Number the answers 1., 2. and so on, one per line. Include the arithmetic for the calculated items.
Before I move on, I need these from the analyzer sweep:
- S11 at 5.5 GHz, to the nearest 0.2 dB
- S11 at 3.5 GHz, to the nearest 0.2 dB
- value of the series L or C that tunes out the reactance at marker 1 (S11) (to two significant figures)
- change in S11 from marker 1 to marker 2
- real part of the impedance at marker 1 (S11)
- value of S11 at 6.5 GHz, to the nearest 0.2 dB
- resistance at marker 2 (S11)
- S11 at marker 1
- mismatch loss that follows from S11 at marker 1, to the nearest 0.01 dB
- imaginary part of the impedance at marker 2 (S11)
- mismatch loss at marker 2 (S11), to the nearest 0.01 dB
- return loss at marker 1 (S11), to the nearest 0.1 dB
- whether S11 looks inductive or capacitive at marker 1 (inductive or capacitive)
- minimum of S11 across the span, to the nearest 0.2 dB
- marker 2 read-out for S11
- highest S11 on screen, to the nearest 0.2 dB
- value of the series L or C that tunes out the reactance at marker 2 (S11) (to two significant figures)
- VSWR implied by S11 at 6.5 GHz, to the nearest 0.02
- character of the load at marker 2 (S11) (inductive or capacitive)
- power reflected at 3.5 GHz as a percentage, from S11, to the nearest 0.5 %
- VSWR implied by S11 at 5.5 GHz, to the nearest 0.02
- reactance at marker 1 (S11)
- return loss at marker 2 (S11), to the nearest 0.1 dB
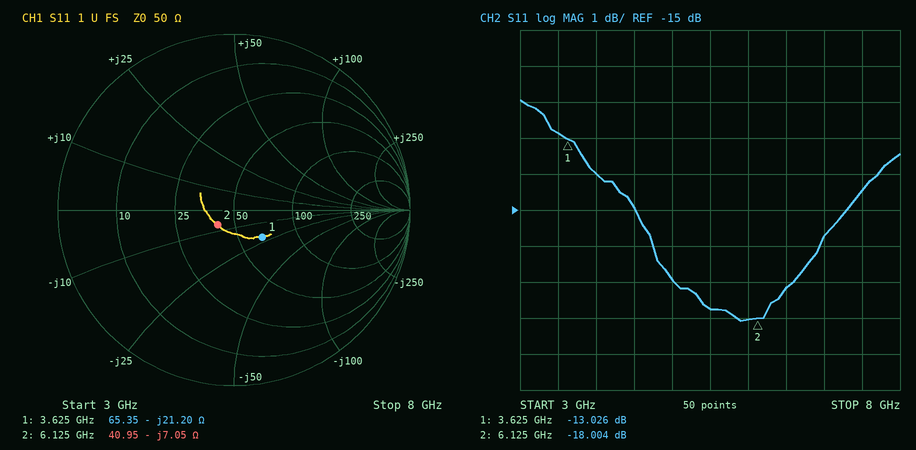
1. -17.8 dB
2. -12.8 dB
3. L = 21.2 Ω/(2π × 3.625 GHz) ≈ 931 pH, so 930 pH to two significant figures
4. -18.004 − (-13.026) = -4.978 dB
5. 65.35 Ω
6. -17.2 dB
7. 40.95 Ω
8. -13.026 dB
9. −10 log10(1 − 10^(-13.026/10)) ≈ 0.22 dB
10. -7.05 Ω
11. −10 log10(1 − 10^(-18.004/10)) ≈ 0.07 dB
12. 13.0 dB
13. capacitive
14. -18.0 dB
15. -18.004 dB
16. -12.0 dB
17. L = 7.05 Ω/(2π × 6.125 GHz) ≈ 183 pH, so 180 pH to two significant figures
18. |Γ| = 10^(-17.2/20) = 0.1380; VSWR = (1 + 0.1380)/(1 − 0.1380) ≈ 1.32
19. capacitive
20. 10^(-12.8/10) ≈ 5.25 %, so 5.0 % to the nearest 0.5 %
21. |Γ| = 10^(-17.8/20) = 0.1288; VSWR = (1 + 0.1288)/(1 − 0.1288) ≈ 1.30
22. -21.20 Ω
23. 18.0 dB
